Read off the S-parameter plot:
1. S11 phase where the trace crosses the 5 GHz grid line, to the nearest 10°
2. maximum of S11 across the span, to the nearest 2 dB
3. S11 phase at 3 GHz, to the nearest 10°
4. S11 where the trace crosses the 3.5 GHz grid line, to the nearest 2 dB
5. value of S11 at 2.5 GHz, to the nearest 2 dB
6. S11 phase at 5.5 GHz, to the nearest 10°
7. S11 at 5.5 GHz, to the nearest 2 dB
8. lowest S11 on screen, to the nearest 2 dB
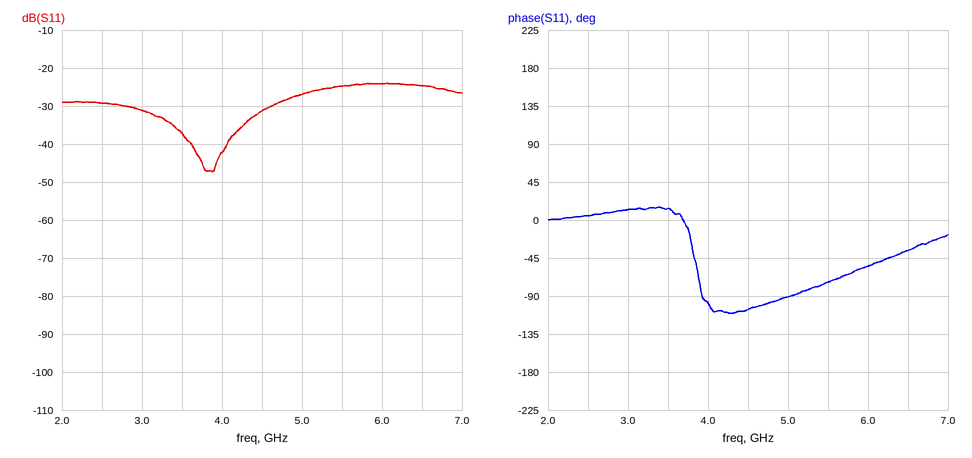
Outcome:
-90°
-24 dB
10°
-38 dB
-30 dB
-70°
-24 dB
-48 dB
